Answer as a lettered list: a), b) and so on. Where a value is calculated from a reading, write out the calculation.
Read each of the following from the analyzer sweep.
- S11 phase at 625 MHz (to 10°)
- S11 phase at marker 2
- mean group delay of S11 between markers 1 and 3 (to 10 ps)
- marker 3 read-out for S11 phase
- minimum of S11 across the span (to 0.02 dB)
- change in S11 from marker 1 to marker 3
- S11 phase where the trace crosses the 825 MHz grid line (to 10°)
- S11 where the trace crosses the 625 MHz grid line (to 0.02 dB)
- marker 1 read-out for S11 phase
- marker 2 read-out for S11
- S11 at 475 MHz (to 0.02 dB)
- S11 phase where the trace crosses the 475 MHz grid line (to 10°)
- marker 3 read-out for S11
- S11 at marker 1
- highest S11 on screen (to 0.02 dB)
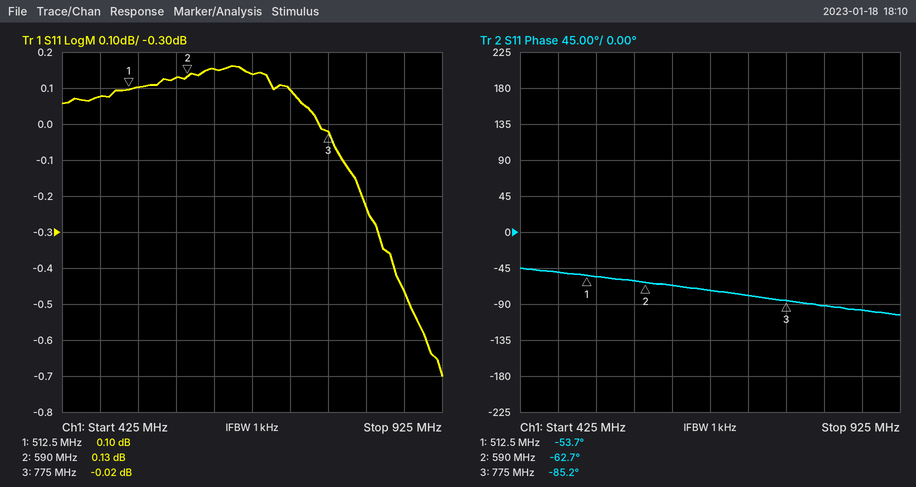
a) -70°
b) -62.7°
c) −(-85.2° − (-53.7°))/(360° × 262.5 MHz) ≈ 333 ps, so 330 ps to the nearest 10 ps
d) -85.2°
e) -0.70 dB
f) -0.02 − (0.1) = -0.12 dB
g) -90°
h) 0.16 dB
i) -53.7°
j) 0.13 dB
k) 0.08 dB
l) -50°
m) -0.02 dB
n) 0.10 dB
o) 0.16 dB
